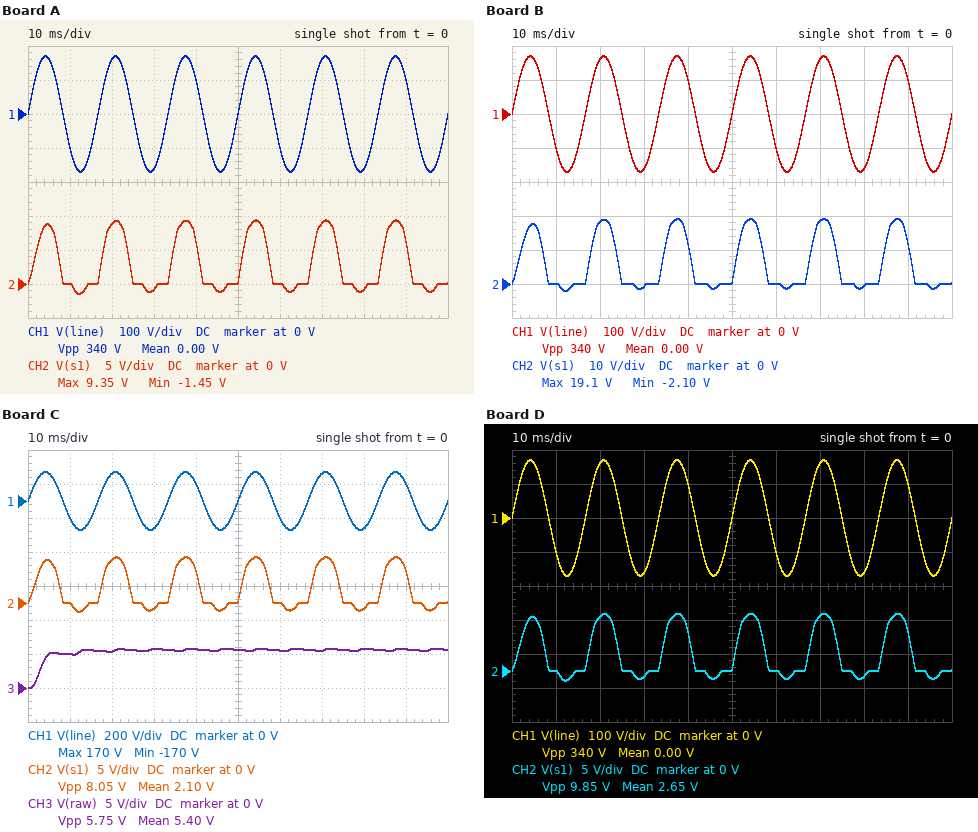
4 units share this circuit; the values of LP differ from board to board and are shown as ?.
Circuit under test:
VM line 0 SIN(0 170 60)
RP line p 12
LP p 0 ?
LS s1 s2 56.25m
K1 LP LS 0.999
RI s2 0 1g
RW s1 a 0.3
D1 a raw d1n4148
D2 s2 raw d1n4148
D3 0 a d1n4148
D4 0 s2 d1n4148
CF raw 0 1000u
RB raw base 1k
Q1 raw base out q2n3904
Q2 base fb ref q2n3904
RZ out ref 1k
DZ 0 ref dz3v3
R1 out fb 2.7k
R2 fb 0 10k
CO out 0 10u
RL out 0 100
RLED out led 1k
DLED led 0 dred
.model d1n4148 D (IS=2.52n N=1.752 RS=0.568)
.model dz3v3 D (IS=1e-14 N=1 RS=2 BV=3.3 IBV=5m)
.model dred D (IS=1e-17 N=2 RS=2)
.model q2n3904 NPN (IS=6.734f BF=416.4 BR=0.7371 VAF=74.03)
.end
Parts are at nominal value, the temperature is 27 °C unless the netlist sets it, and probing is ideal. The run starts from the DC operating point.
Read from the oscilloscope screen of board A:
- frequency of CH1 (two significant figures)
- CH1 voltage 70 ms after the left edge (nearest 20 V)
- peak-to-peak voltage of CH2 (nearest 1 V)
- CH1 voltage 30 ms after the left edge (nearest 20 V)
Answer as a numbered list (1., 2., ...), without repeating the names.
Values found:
1. 60 Hz
2. 160 V
3. 11 V
4. -160 V
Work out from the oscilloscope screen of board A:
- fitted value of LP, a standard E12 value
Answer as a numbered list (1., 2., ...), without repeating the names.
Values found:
1. 15 H
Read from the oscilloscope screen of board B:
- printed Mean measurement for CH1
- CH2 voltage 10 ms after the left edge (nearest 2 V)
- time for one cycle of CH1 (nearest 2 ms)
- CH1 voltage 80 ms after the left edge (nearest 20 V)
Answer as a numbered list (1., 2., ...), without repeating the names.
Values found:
1. 0.00 V
2. 0 V
3. 16 ms
4. -160 V
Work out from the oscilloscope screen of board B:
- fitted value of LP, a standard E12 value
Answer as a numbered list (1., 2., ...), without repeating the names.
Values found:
1. 3.9 H
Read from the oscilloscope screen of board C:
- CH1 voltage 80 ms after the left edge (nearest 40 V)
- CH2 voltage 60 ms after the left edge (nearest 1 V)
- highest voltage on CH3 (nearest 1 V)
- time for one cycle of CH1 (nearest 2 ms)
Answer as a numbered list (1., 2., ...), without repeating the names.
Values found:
1. -160 V
2. 0 V
3. 6 V
4. 16 ms
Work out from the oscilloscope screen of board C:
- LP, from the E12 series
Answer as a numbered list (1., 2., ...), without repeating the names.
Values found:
1. 27 H
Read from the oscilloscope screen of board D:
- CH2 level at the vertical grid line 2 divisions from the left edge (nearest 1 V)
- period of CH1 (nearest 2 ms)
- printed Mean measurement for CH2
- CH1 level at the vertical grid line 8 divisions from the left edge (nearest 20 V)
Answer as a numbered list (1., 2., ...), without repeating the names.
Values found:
1. 8 V
2. 16 ms
3. 2.65 V
4. -160 V
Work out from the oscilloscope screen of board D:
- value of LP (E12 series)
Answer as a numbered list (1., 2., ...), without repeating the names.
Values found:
1. 18 H
